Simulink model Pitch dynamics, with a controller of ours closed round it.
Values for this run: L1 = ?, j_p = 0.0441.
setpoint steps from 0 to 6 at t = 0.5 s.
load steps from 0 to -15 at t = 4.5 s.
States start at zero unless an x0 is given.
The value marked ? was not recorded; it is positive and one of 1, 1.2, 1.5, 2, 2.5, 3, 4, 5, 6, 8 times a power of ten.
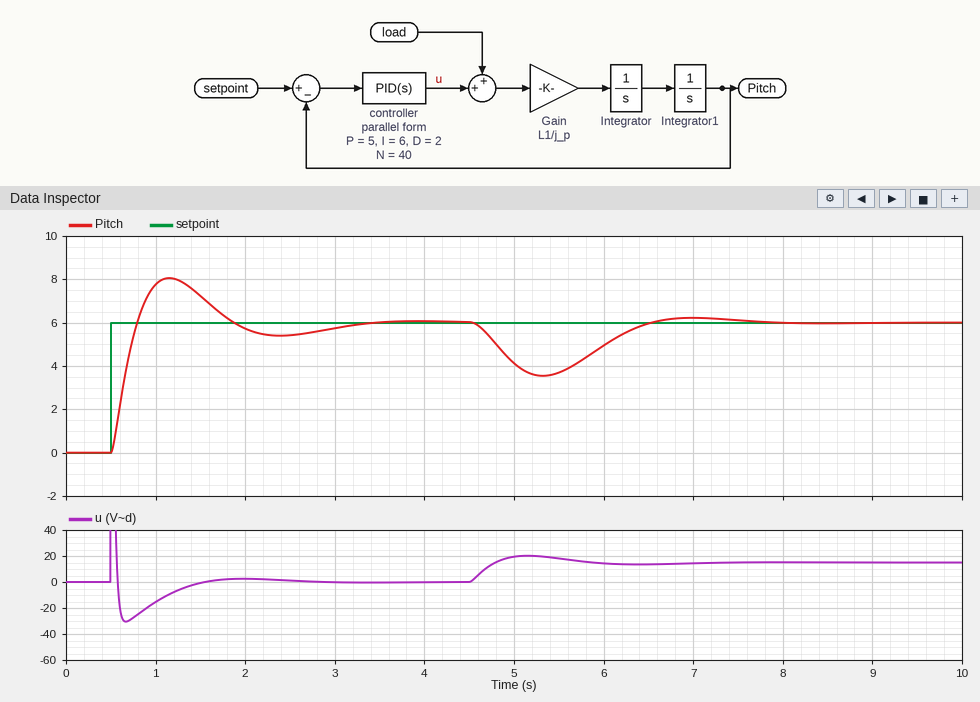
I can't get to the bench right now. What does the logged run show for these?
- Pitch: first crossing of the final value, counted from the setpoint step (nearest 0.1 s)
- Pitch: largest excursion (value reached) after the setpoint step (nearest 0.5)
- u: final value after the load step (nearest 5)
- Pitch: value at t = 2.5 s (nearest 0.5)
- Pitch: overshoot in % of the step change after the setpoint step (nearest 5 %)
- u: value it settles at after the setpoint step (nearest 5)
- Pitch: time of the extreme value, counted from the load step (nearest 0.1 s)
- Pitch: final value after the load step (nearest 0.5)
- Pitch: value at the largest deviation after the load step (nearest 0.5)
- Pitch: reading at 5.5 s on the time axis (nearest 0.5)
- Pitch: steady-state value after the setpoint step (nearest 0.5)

0.3 s
8.0
15
5.5
35 %
0
0.8 s
6.0
3.5
3.5
6.0
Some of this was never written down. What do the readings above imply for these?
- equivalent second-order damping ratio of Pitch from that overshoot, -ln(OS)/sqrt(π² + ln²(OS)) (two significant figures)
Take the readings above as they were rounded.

0.32
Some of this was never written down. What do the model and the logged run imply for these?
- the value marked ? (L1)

0.1
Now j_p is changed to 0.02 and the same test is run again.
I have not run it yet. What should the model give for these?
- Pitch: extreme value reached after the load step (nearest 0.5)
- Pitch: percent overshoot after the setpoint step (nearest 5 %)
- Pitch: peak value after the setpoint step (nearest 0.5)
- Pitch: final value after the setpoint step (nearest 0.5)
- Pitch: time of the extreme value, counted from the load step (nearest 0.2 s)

4.0
20 %
7.0
6.0
0.6 s
